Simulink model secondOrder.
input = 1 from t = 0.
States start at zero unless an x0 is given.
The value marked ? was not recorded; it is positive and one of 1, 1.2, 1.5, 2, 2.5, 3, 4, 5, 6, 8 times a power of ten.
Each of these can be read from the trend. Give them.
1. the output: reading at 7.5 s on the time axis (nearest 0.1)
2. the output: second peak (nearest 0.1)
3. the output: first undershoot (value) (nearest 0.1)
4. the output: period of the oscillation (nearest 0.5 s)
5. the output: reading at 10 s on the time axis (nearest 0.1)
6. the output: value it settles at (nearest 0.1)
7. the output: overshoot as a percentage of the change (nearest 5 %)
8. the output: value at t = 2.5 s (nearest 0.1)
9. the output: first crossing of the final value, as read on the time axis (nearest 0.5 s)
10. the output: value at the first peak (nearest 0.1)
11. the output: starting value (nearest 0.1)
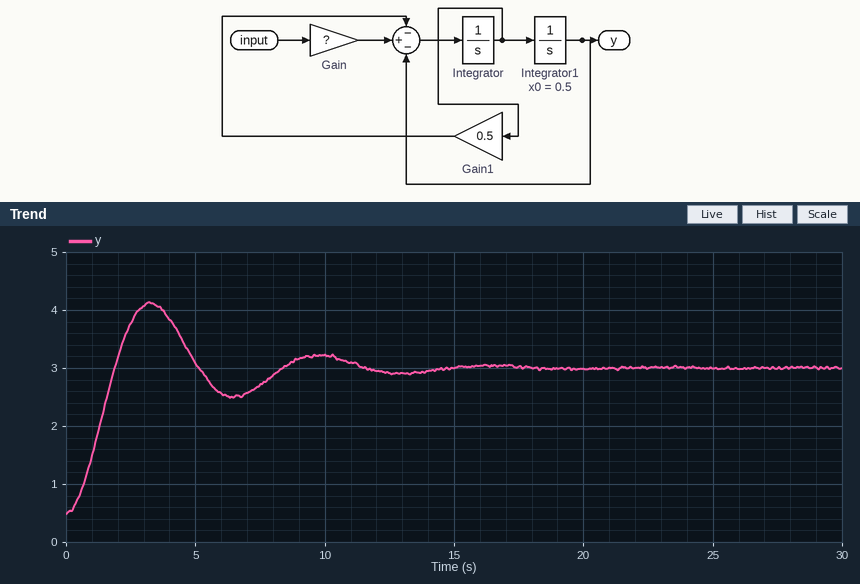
2.7
3.2
2.5
6.5 s
3.2
3.0
45 %
3.8
2.0 s
4.1
0.5
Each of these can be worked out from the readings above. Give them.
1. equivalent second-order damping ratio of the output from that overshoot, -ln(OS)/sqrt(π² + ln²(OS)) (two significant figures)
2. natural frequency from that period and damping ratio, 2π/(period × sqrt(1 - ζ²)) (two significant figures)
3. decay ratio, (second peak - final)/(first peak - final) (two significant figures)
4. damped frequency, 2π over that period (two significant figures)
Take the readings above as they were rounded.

0.25
1.00 rad/s
0.18
0.97 rad/s
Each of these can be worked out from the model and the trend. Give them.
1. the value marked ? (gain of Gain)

3
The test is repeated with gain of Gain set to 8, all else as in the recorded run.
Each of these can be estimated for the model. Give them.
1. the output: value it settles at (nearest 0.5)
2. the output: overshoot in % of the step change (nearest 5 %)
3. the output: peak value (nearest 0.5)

8.0
45 %
11.5
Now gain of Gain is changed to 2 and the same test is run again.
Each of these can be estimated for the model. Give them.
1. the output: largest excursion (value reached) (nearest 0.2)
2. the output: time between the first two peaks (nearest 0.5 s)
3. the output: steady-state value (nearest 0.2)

2.6
6.5 s
2.0
